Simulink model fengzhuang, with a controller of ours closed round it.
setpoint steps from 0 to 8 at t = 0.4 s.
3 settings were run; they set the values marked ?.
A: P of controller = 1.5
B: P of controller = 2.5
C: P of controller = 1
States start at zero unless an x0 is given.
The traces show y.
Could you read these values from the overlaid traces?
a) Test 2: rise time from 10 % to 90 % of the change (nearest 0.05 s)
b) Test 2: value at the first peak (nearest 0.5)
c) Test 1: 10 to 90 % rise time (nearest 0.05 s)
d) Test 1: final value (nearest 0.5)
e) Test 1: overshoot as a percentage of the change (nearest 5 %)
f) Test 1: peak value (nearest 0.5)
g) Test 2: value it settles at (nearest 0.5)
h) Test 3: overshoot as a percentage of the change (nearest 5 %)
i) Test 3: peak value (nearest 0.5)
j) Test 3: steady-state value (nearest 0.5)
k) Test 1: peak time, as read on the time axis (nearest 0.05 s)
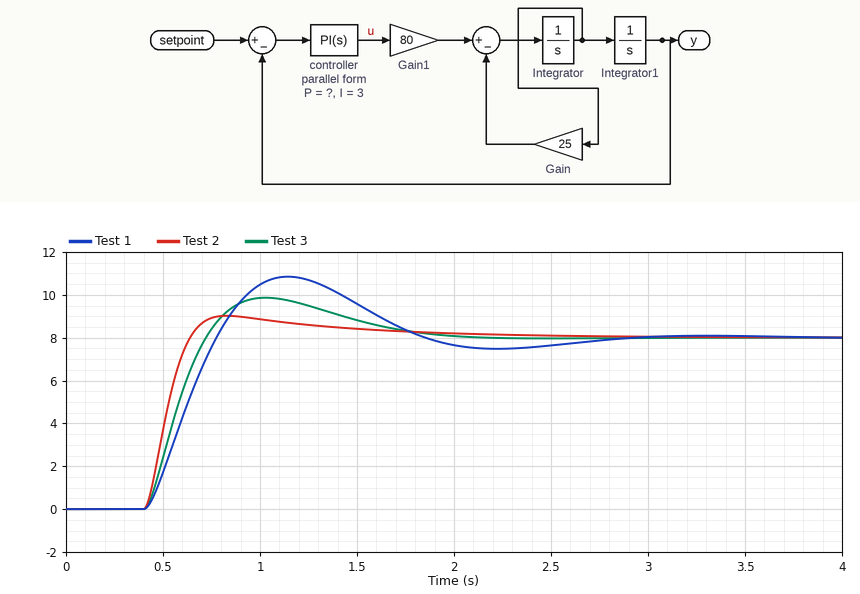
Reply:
0.15 s
9.0
0.25 s
8.0
35 %
11.0
8.0
25 %
10.0
8.0
1.15 s
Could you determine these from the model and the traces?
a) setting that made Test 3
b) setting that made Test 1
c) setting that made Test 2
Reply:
A
C
B
